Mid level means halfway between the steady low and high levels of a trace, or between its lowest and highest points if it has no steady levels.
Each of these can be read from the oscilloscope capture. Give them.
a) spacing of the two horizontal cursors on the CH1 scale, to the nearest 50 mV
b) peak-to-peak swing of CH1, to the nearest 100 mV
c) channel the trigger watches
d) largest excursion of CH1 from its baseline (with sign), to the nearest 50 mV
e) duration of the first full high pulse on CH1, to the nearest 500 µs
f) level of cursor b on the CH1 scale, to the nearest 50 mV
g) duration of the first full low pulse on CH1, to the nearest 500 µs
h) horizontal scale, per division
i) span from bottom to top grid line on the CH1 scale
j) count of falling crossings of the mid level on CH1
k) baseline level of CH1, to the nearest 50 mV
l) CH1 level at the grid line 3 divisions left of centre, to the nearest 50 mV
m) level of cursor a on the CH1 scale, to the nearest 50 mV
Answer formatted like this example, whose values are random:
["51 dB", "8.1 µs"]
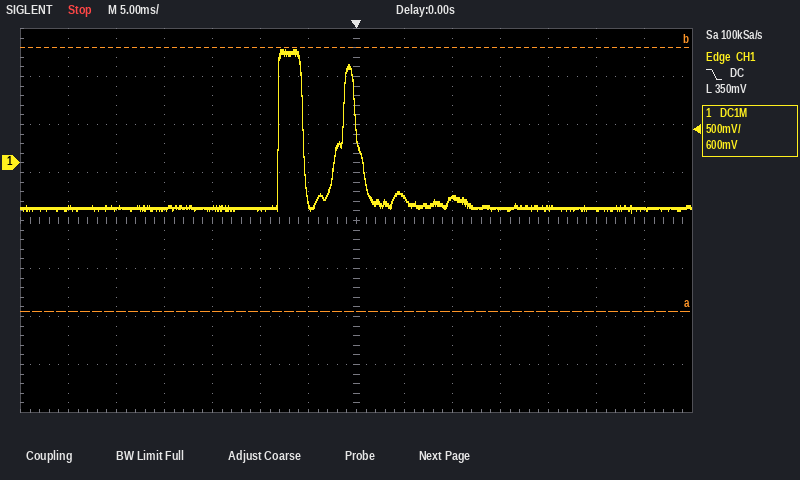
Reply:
["2.75 V", "1.70 V", "CH1", "+1.65 V", "2.5 ms", "1.20 V", "4.0 ms", "5 ms", "4 V", "2", "-450 mV", "-450 mV", "-1.55 V"]
